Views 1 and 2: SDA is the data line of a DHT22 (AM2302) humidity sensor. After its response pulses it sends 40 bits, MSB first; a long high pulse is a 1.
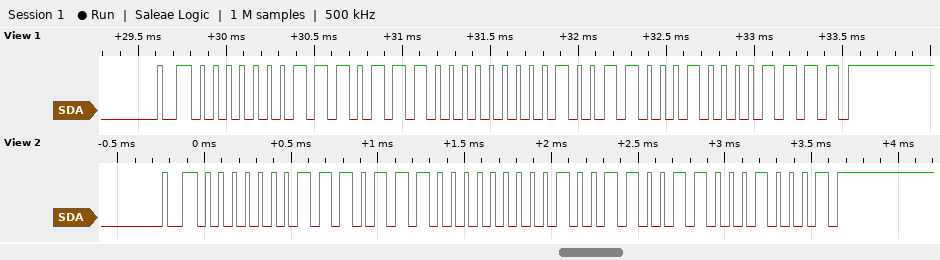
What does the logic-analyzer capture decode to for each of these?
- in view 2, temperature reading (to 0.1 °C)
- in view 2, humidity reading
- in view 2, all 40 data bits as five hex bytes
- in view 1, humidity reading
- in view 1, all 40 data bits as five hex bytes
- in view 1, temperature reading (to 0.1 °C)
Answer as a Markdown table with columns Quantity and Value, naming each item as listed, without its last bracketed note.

| Quantity | Value |
|---|---|
| in view 2, temperature reading | 30.7 °C |
| in view 2, humidity reading | 47.6 % |
| in view 2, all 40 data bits as five hex bytes | 01 DC 01 33 11 |
| in view 1, humidity reading | 47.6 % |
| in view 1, all 40 data bits as five hex bytes | 01 DC 01 31 0F |
| in view 1, temperature reading | 30.5 °C |
